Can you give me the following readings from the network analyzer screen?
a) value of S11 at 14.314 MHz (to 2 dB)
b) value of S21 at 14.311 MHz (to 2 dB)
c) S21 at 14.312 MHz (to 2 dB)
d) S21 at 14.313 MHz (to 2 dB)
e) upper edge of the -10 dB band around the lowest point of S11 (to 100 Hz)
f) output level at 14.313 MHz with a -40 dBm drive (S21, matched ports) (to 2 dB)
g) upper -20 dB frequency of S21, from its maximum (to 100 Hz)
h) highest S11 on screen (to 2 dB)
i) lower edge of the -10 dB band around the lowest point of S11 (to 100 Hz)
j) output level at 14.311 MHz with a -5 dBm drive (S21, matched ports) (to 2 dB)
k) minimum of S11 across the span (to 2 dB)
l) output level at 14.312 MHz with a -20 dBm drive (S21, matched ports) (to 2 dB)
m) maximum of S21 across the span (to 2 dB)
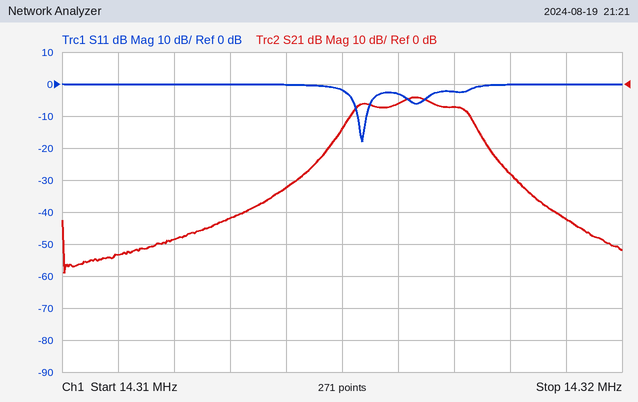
0 dB
-54 dB
-48 dB
-42 dB
14.3154 MHz
-82 dBm
14.3178 MHz
0 dB
14.3153 MHz
-58 dBm
-18 dB
-68 dBm
-4 dB
